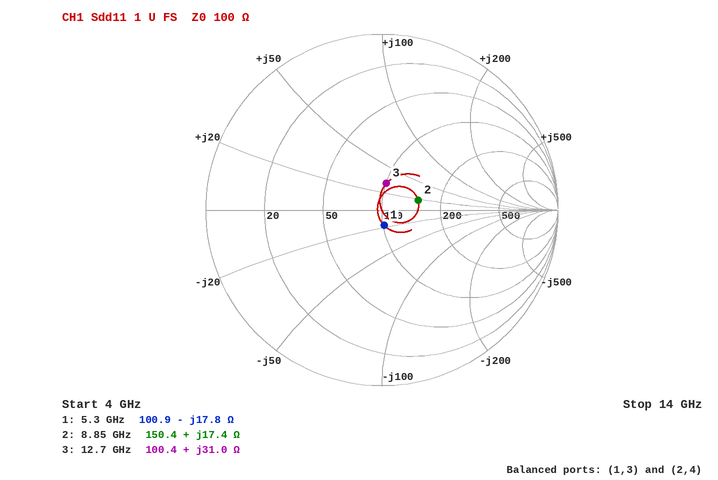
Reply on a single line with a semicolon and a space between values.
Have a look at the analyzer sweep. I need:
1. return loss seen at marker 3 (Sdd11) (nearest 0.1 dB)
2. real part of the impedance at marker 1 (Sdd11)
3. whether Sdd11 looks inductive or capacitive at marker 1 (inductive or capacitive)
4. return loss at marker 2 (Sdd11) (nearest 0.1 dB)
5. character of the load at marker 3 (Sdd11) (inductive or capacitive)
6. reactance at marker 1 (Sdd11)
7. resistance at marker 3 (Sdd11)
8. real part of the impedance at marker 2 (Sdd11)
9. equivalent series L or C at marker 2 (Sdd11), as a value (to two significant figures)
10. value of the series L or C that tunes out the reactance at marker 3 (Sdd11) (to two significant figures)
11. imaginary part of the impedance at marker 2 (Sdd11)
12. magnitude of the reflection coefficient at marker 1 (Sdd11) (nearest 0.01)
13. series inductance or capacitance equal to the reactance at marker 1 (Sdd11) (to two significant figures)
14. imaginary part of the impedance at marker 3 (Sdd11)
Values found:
16.3 dB; 100.9 Ω; capacitive; 13.5 dB; inductive; -17.8 Ω; 100.4 Ω; 150.4 Ω; 310 pH; 400 fF; +17.4 Ω; 0.09; 1.7 pF; +31.0 Ω
